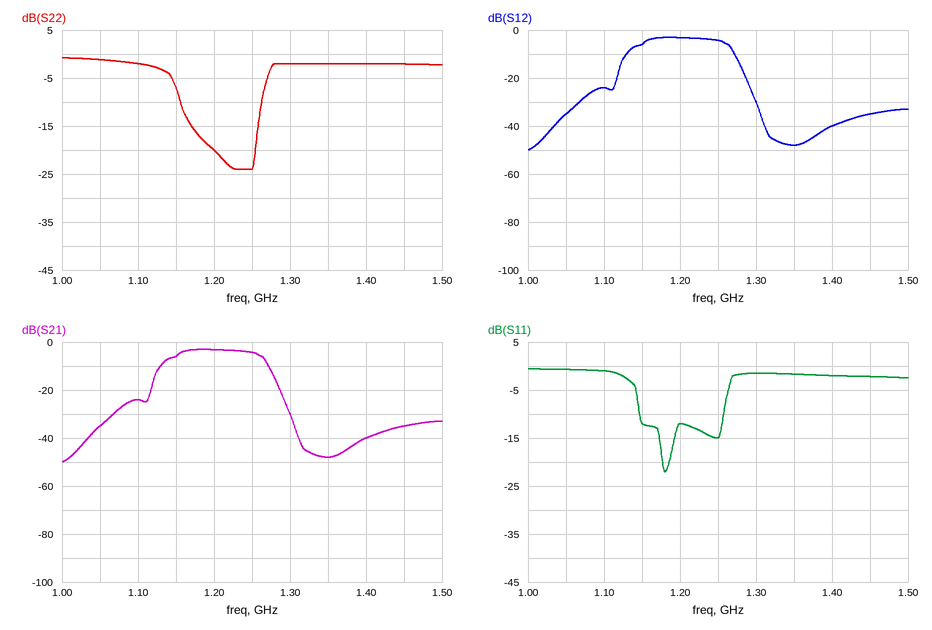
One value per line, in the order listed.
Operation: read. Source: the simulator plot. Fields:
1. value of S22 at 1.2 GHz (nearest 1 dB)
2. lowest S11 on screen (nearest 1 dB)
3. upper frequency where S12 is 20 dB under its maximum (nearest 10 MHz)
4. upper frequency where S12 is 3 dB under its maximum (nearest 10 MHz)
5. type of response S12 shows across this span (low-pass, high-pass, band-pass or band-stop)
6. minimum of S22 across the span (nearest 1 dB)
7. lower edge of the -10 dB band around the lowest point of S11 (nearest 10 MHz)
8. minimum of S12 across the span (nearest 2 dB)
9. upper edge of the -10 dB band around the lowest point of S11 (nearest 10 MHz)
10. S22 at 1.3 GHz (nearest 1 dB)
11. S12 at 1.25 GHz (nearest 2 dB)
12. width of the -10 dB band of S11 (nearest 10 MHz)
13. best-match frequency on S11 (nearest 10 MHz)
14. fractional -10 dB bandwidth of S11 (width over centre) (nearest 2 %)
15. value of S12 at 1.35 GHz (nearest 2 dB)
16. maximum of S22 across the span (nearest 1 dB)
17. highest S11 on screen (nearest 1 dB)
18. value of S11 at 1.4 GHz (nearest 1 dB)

-20 dB
-22 dB
1.29 GHz
1.26 GHz
band-pass
-24 dB
1.15 GHz
-50 dB
1.26 GHz
-2 dB
-4 dB
110 MHz
1.18 GHz
10 %
-48 dB
-1 dB
-1 dB
-2 dB
